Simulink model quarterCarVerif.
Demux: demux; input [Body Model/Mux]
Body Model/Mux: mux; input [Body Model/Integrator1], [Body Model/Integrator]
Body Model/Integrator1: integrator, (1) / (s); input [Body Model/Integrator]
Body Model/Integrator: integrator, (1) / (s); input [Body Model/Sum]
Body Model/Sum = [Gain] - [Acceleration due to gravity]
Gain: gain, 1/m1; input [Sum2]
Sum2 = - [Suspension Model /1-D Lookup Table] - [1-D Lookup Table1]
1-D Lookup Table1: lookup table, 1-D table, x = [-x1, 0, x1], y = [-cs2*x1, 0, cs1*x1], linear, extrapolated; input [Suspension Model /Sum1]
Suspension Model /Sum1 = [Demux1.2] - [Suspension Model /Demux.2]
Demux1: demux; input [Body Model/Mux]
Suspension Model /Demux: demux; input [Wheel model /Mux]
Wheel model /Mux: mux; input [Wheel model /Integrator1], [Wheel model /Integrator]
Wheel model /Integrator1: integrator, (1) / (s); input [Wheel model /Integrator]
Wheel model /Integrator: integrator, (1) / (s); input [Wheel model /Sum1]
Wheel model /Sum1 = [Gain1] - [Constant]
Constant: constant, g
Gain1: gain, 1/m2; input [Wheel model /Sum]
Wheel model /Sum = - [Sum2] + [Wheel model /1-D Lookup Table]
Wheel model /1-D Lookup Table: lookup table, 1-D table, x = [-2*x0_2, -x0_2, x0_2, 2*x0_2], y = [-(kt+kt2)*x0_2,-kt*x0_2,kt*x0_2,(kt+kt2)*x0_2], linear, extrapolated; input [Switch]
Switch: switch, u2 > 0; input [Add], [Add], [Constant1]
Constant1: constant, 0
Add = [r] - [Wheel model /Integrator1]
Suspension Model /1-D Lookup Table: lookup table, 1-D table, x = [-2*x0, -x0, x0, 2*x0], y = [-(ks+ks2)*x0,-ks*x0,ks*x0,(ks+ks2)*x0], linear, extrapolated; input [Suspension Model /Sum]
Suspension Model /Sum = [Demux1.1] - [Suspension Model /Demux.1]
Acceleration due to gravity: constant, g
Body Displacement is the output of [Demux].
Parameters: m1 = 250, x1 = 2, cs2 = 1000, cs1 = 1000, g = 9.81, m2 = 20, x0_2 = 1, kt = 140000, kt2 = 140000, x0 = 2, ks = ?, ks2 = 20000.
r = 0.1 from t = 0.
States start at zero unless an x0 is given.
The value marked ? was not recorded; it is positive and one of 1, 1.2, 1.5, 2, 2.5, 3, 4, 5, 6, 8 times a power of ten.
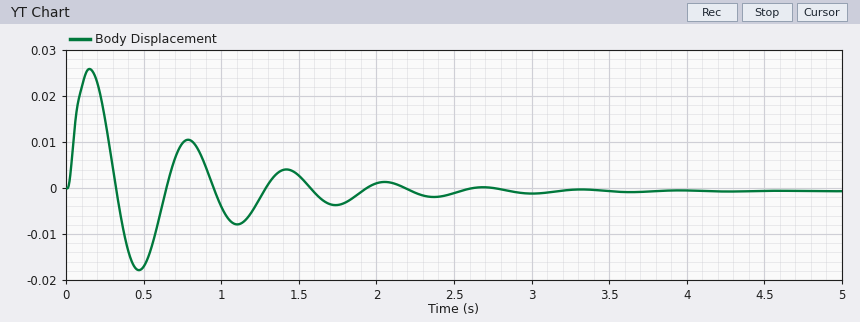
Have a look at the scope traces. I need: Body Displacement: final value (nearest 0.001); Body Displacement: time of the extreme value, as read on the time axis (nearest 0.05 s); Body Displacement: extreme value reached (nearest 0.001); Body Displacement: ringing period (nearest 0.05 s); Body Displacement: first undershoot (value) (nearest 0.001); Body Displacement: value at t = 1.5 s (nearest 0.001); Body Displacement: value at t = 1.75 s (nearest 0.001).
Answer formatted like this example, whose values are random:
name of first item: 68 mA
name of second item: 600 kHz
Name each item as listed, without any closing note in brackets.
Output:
Body Displacement: final value: -0.001
Body Displacement: time of the extreme value, as read on the time axis: 0.15 s
Body Displacement: extreme value reached: 0.026
Body Displacement: ringing period: 0.65 s
Body Displacement: first undershoot (value): -0.018
Body Displacement: value at t = 1.5 s: 0.003
Body Displacement: value at t = 1.75 s: -0.004
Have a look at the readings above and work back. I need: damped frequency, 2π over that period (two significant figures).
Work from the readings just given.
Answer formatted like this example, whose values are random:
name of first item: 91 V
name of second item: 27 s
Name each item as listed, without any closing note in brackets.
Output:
damped frequency, 2π over that period: 9.7 rad/s
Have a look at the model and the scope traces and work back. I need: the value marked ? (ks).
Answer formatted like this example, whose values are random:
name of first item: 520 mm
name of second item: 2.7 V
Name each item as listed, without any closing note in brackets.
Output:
the value marked ?: 30000
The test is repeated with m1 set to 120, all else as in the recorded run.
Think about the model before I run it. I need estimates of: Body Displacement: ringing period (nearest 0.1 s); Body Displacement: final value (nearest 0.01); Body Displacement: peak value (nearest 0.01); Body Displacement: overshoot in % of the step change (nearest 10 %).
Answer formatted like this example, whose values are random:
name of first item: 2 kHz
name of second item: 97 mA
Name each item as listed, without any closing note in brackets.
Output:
Body Displacement: ringing period: 0.4 s
Body Displacement: final value: 0.05
Body Displacement: peak value: 0.10
Body Displacement: overshoot in % of the step change: 100 %
